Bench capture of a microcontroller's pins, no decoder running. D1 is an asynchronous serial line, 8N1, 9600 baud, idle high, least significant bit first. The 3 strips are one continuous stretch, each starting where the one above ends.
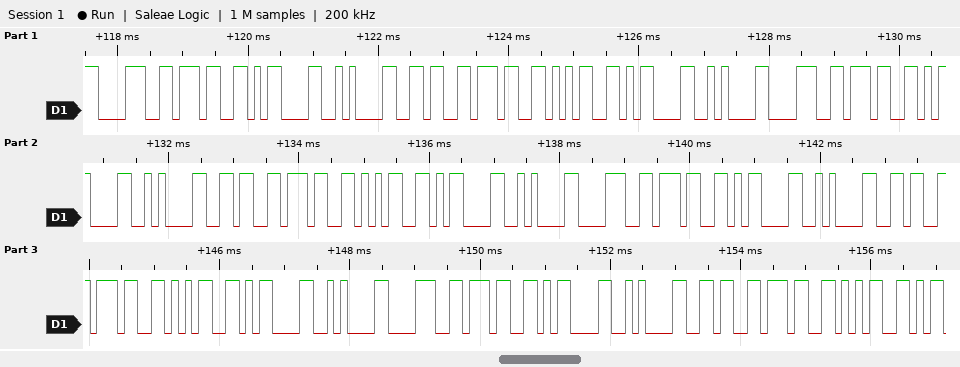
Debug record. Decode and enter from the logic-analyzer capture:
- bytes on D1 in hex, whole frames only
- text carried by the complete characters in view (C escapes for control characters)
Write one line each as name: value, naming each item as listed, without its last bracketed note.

bytes on D1 in hex, whole frames only: 38 37 0D 0A 36 37 35 0D 0A 38 37 0D 0A 36 37 35 0D 0A 38 37 0D 0A 36 37 35 0D 0A 38 37 0D 0A 36 37 35
text carried by the complete characters in view: "87\r\n675\r\n87\r\n675\r\n87\r\n675\r\n87\r\n675"
